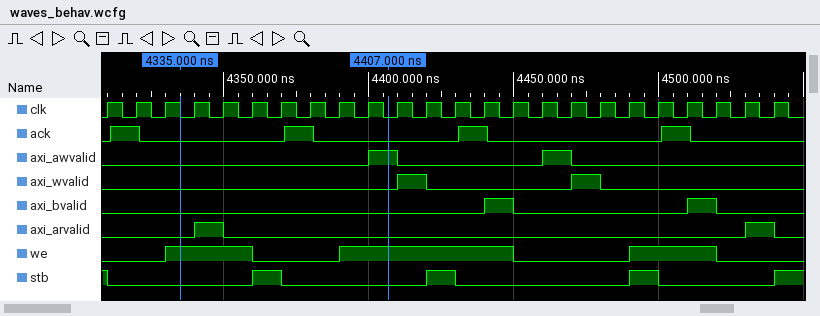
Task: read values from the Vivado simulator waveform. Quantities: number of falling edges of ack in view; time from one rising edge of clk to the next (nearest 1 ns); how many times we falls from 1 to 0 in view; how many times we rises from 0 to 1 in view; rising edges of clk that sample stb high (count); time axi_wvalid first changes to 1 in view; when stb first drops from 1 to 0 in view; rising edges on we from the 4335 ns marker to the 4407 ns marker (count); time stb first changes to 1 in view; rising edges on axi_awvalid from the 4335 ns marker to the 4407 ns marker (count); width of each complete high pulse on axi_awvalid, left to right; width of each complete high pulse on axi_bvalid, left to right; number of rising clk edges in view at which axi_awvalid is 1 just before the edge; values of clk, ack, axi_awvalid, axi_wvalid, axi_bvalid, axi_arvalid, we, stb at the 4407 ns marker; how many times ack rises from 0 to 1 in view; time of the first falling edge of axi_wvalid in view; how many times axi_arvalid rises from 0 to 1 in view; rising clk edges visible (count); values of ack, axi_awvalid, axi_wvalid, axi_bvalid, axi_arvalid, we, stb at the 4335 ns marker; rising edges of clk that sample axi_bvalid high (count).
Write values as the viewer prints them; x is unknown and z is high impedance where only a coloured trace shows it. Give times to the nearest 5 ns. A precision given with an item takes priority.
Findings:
4
10 ns
3
3
4
4410 ns
4310 ns
1
4360 ns
1
10 ns, 10 ns
10 ns, 10 ns
2
clk=0, ack=0, axi_awvalid=1, axi_wvalid=0, axi_bvalid=0, axi_arvalid=0, we=1, stb=0
4
4420 ns
2
24
ack=0, axi_awvalid=0, axi_wvalid=0, axi_bvalid=0, axi_arvalid=0, we=1, stb=0
2
